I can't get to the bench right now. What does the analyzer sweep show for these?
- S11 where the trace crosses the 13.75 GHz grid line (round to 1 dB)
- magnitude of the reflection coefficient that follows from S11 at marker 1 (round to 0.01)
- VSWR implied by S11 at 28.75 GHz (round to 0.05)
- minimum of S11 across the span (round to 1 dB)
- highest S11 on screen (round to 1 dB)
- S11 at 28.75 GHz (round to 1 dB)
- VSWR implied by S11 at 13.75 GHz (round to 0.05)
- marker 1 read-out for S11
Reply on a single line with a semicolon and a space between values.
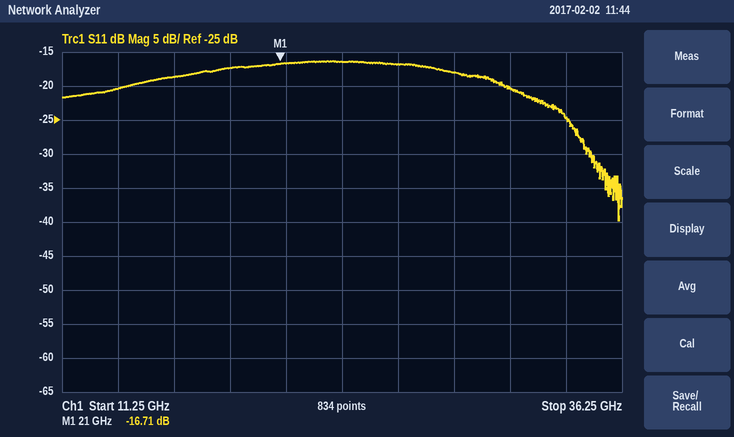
-20 dB; 0.15; 1.30; -40 dB; -16 dB; -18 dB; 1.20; -16.71 dB
